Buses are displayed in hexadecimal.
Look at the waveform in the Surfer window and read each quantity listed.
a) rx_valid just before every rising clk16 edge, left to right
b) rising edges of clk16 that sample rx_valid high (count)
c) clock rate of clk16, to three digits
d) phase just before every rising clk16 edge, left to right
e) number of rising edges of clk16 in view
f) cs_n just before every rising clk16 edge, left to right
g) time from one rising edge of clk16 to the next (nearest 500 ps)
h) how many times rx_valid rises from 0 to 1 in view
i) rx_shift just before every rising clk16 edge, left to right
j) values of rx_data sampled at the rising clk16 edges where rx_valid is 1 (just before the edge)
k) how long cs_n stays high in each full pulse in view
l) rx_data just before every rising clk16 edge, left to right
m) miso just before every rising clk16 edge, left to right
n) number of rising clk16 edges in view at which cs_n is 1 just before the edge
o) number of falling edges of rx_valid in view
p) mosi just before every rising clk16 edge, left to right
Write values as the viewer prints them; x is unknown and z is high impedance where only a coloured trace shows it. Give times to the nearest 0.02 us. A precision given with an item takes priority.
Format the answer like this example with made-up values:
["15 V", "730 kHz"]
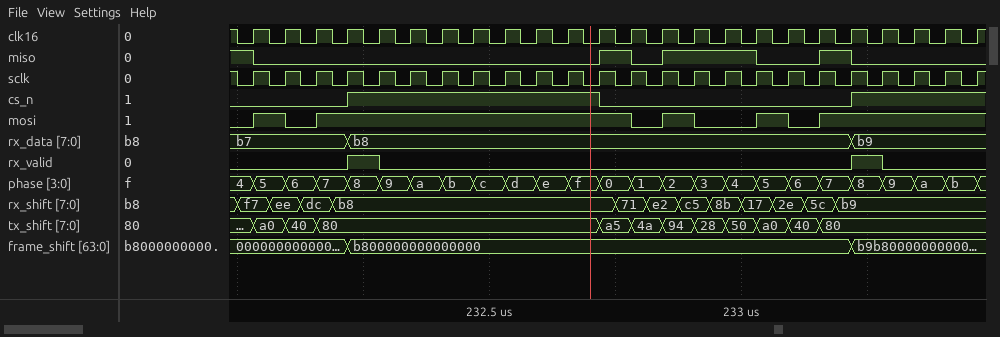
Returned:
["0 0 0 0 1 0 0 0 0 0 0 0 0 0 0 0 0 0 0 0 1 0 0 0", "2", "16.0 MHz", "4, 5, 6, 7, 8, 9, a, b, c, d, e, f, 0, 1, 2, 3, 4, 5, 6, 7, 8, 9, a, b", "24", "0 0 0 0 1 1 1 1 1 1 1 1 0 0 0 0 0 0 0 0 1 1 1 1", "62500 ps", "2", "f7, ee, dc, b8, b8, b8, b8, b8, b8, b8, b8, b8, 71, e2, c5, 8b, 17, 2e, 5c, b9, b9, b9, b9, b9", "b8, b9", "0.5 us", "b7, b7, b7, b7, b8, b8, b8, b8, b8, b8, b8, b8, b8, b8, b8, b8, b8, b8, b8, b8, b9, b9, b9, b9", "1 0 0 0 0 0 0 0 0 0 0 0 1 0 1 1 1 0 0 1 0 0 0 0", "12", "2", "0 1 0 1 1 1 1 1 1 1 1 1 1 0 1 0 0 1 0 1 1 1 1 1"]
